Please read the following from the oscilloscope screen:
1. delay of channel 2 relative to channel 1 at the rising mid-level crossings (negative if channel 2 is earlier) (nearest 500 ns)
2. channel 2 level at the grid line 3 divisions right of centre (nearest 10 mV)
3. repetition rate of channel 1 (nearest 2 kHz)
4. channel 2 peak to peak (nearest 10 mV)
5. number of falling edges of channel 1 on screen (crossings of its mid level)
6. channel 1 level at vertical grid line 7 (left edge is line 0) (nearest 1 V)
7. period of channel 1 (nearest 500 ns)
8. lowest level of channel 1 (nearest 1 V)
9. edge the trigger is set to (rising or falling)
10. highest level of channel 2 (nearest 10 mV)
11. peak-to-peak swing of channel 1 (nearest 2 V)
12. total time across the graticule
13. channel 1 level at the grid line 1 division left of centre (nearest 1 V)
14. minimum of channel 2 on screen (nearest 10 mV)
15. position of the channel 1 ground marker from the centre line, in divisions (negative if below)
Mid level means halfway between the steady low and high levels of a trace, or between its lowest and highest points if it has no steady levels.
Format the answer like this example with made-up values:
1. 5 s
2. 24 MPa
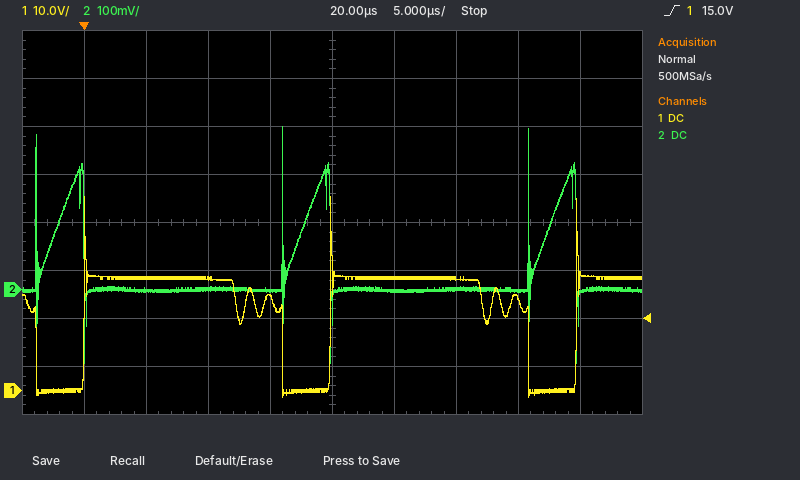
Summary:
1. -2.5 µs
2. 0 mV
3. 50 kHz
4. 490 mV
5. 3
6. 23 V
7. 20.0 µs
8. -1 V
9. rising
10. 340 mV
11. 42 V
12. 50 µs
13. 19 V
14. -150 mV
15. -3.5 div
